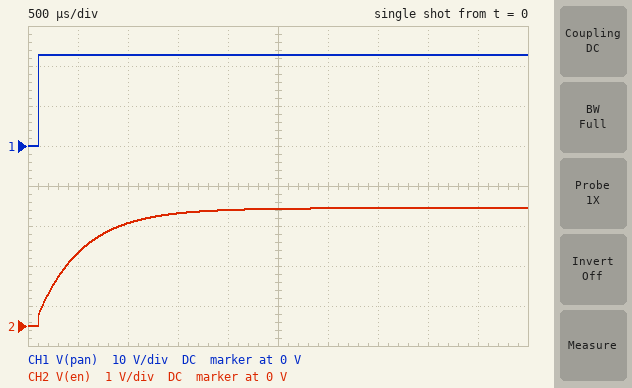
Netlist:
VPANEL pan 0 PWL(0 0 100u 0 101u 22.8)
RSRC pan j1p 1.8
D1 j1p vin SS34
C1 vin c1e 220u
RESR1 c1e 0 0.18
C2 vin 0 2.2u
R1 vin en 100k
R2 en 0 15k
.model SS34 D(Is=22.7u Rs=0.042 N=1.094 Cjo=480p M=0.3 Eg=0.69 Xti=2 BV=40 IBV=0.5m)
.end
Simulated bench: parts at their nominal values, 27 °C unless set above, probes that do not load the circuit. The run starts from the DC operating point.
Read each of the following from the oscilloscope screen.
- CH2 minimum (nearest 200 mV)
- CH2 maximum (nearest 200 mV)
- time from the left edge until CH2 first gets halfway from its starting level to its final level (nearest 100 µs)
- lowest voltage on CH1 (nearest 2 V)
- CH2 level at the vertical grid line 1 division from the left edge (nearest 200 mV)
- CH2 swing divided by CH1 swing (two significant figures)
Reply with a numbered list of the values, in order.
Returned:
1. 0 V
2. 3.0 V
3. 400 µs
4. 0 V
5. 1.8 V
6. 0.13
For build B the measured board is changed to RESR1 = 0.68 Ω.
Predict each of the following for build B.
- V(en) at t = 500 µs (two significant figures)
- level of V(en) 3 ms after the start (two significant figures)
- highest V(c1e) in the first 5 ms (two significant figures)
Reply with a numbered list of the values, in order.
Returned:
1. 1.9 V
2. 2.9 V
3. 6.0 V
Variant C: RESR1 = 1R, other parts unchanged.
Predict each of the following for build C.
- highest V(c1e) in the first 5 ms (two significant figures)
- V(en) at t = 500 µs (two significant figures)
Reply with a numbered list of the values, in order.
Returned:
1. 7.8 V
2. 1.9 V
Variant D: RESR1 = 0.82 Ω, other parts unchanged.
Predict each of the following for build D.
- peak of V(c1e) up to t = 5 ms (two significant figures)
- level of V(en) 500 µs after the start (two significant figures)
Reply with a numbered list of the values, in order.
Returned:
1. 6.8 V
2. 1.9 V
